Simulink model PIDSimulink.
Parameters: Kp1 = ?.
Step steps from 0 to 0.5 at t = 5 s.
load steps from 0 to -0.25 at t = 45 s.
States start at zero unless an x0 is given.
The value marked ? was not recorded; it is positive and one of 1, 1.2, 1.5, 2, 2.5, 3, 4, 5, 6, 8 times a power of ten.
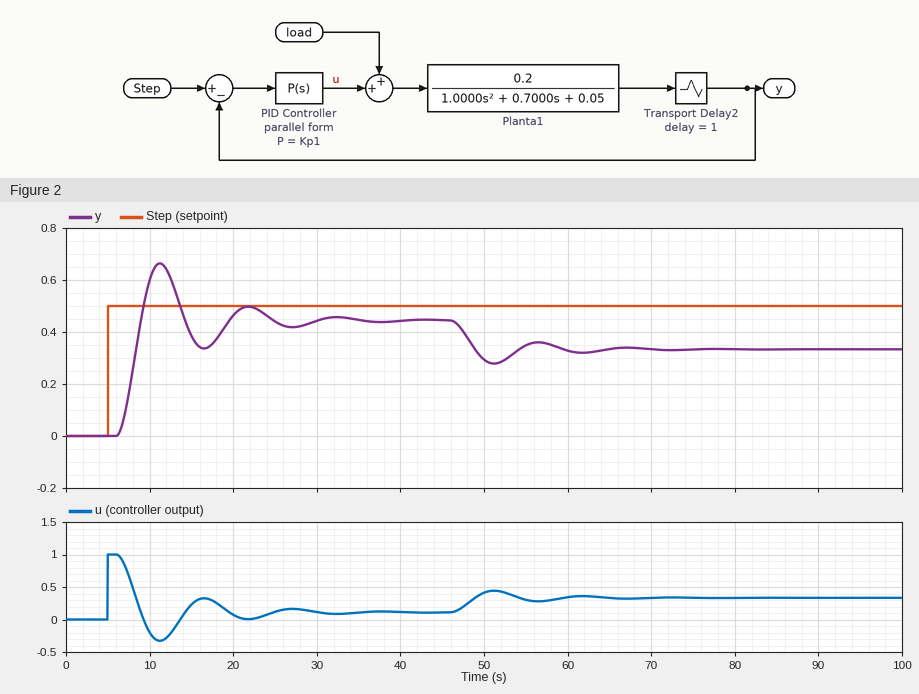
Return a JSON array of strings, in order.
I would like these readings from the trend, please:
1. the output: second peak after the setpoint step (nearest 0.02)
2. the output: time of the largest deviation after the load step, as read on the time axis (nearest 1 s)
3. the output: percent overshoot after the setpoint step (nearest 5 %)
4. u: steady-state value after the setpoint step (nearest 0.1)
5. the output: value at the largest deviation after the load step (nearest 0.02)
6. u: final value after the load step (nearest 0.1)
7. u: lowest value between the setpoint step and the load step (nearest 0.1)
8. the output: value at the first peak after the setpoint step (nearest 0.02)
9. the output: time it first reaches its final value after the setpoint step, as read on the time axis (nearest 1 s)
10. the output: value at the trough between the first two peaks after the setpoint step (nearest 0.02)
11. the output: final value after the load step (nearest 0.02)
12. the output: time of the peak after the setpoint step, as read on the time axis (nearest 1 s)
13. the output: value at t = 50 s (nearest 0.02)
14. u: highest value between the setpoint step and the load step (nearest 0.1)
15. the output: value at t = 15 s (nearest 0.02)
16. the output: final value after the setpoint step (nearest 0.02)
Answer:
["0.50", "51 s", "50 %", "0.1", "0.28", "0.3", "-0.3", "0.66", "9 s", "0.34", "0.34", "11 s", "0.30", "1.0", "0.38", "0.44"]
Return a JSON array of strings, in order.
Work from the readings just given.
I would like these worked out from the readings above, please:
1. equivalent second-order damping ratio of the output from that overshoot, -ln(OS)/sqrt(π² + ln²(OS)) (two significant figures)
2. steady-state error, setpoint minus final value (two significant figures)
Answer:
["0.22", "0.060"]
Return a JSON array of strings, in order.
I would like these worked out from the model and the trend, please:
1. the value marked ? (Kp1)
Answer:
["2"]
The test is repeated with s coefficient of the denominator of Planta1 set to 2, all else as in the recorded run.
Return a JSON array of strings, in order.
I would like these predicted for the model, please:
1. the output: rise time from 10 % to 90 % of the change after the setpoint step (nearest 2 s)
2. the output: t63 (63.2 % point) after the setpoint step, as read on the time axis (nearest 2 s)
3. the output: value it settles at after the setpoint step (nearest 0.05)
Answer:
["6 s", "10 s", "0.45"]
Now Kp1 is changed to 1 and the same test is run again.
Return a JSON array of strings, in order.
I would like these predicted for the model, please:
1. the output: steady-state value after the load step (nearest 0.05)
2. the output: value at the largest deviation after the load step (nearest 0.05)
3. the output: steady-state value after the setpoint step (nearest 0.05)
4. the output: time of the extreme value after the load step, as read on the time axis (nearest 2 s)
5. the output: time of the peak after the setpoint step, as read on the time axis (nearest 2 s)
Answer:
["0.20", "0.15", "0.40", "54 s", "14 s"]
